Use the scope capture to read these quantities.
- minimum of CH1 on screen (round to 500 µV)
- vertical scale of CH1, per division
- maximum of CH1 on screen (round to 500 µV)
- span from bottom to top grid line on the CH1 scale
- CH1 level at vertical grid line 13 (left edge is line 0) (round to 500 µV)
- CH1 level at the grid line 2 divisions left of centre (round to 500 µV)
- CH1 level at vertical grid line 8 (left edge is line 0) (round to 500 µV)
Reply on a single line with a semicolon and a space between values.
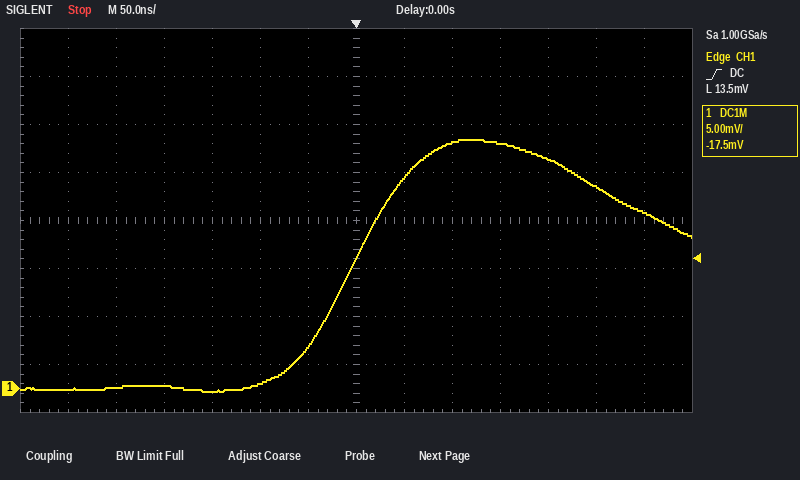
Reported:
-500 µV; 5 mV; 26.0 mV; 40 mV; 18.5 mV; 500 µV; 22.0 mV
